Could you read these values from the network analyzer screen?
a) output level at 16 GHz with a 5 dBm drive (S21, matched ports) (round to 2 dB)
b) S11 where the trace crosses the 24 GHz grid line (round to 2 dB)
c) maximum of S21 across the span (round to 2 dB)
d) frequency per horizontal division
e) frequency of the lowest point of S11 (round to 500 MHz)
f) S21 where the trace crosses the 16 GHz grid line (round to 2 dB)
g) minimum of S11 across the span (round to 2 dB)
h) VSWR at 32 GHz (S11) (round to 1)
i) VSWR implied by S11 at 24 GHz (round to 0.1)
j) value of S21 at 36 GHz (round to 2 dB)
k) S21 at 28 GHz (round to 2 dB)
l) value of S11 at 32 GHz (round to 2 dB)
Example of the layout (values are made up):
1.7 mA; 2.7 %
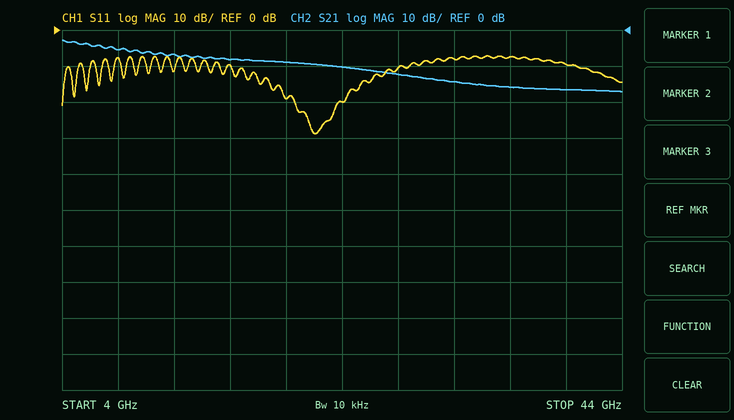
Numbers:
-4 dBm; -20 dB; -2 dB; 4 GHz; 22.0 GHz; -8 dB; -28 dB; 2; 1.2; -16 dB; -12 dB; -8 dB
